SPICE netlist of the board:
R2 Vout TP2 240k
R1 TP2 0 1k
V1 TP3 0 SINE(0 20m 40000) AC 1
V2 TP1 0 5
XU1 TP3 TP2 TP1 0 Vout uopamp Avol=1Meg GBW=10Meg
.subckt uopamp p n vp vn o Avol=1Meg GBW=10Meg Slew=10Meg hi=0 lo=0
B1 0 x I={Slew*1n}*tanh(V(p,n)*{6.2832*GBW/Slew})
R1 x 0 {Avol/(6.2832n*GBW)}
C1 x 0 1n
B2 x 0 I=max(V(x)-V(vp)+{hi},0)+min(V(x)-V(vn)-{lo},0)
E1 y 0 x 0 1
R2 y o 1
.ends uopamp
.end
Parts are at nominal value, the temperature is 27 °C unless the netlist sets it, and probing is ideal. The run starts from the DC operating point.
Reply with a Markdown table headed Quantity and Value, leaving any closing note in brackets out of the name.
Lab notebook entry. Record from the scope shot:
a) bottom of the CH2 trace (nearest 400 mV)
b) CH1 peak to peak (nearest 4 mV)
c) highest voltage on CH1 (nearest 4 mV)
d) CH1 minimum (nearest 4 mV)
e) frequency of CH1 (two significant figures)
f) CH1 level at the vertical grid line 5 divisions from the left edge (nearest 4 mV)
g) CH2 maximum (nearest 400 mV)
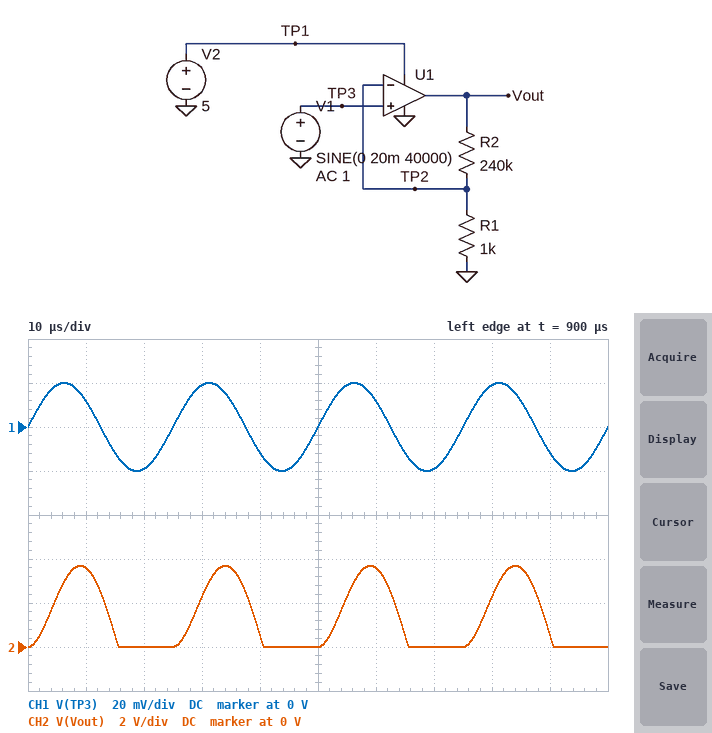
| Quantity | Value |
|---|---|
| bottom of the CH2 trace | 0 V |
| CH1 peak to peak | 40 mV |
| highest voltage on CH1 | 20 mV |
| CH1 minimum | -20 mV |
| frequency of CH1 | 40 kHz |
| CH1 level at the vertical grid line 5 divisions from the left edge | 0 V |
| CH2 maximum | 3.6 V |
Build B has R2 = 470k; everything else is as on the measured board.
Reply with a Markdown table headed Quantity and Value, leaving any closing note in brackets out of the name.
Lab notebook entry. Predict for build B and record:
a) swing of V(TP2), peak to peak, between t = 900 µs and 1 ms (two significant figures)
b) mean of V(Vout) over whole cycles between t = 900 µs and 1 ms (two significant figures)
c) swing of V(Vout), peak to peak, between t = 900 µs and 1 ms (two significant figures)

| Quantity | Value |
|---|---|
| swing of V(TP2), peak to peak, between t = 900 µs and 1 ms | 11 mV |
| mean of V(Vout) over whole cycles between t = 900 µs and 1 ms | 2.0 V |
| swing of V(Vout), peak to peak, between t = 900 µs and 1 ms | 5.0 V |
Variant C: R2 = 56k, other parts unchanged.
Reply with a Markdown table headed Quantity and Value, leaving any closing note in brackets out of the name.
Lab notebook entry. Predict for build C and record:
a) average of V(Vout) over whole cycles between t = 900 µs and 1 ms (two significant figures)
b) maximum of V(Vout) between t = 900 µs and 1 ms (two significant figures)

| Quantity | Value |
|---|---|
| average of V(Vout) over whole cycles between t = 900 µs and 1 ms | 360 mV |
| maximum of V(Vout) between t = 900 µs and 1 ms | 1.1 V |
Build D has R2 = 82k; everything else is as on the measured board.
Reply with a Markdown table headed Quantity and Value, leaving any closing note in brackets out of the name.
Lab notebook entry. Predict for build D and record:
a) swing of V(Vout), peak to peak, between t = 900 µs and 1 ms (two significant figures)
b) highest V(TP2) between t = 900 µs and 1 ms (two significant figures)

| Quantity | Value |
|---|---|
| swing of V(Vout), peak to peak, between t = 900 µs and 1 ms | 1.6 V |
| highest V(TP2) between t = 900 µs and 1 ms | 19 mV |
